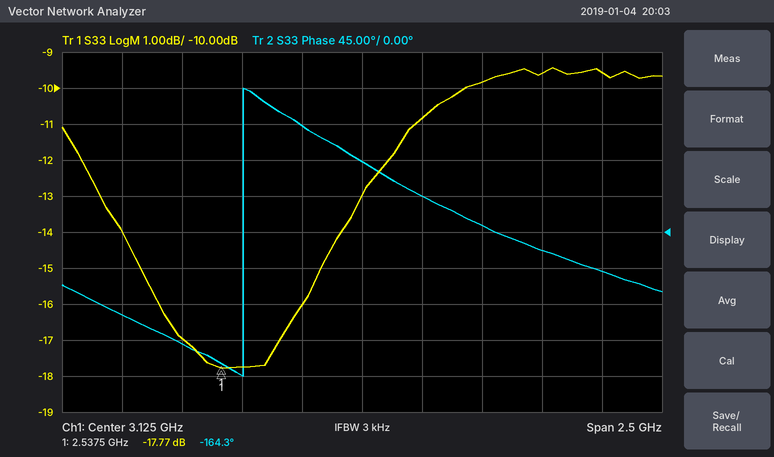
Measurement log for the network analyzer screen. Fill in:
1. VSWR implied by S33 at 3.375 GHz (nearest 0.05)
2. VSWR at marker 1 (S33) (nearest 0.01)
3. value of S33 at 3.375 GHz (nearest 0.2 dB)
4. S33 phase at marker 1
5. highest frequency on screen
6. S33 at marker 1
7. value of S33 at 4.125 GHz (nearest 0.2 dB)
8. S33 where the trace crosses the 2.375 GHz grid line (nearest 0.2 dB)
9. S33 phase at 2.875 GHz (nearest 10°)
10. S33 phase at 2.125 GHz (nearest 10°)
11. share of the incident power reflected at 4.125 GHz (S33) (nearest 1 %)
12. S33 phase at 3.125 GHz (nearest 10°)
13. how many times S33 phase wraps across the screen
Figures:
1.80
1.30
-10.8 dB
-164.3°
4.375 GHz
-17.77 dB
-9.6 dB
-17.0 dB
130°
-100°
11 %
90°
1
